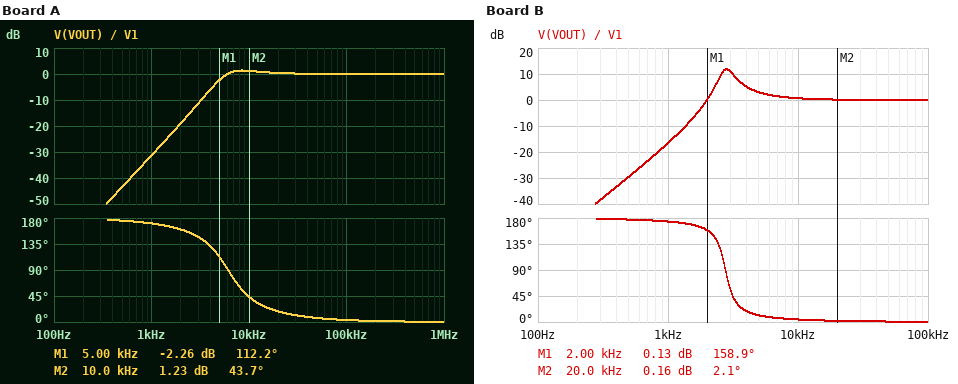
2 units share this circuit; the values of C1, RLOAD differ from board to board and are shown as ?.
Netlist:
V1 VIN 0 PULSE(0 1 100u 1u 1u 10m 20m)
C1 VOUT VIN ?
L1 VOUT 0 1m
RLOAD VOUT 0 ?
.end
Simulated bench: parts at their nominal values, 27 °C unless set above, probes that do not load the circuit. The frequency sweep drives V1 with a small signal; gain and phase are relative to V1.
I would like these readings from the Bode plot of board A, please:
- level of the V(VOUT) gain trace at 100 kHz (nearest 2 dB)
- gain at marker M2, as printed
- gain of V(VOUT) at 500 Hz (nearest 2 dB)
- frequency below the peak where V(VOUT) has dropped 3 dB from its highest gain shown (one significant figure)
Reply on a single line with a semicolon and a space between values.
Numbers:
0 dB; 1.23 dB; -44 dB; 5 kHz
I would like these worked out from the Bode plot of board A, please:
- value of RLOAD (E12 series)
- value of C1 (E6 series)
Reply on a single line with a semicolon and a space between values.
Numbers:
39 Ω; 680 nF
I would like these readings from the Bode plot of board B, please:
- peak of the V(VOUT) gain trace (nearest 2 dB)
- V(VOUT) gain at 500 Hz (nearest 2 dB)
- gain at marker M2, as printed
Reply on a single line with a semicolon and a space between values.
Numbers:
12 dB; -30 dB; 0.16 dB
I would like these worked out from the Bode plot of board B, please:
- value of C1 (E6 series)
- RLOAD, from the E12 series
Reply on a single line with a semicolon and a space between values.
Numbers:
3.3 µF; 68 Ω
